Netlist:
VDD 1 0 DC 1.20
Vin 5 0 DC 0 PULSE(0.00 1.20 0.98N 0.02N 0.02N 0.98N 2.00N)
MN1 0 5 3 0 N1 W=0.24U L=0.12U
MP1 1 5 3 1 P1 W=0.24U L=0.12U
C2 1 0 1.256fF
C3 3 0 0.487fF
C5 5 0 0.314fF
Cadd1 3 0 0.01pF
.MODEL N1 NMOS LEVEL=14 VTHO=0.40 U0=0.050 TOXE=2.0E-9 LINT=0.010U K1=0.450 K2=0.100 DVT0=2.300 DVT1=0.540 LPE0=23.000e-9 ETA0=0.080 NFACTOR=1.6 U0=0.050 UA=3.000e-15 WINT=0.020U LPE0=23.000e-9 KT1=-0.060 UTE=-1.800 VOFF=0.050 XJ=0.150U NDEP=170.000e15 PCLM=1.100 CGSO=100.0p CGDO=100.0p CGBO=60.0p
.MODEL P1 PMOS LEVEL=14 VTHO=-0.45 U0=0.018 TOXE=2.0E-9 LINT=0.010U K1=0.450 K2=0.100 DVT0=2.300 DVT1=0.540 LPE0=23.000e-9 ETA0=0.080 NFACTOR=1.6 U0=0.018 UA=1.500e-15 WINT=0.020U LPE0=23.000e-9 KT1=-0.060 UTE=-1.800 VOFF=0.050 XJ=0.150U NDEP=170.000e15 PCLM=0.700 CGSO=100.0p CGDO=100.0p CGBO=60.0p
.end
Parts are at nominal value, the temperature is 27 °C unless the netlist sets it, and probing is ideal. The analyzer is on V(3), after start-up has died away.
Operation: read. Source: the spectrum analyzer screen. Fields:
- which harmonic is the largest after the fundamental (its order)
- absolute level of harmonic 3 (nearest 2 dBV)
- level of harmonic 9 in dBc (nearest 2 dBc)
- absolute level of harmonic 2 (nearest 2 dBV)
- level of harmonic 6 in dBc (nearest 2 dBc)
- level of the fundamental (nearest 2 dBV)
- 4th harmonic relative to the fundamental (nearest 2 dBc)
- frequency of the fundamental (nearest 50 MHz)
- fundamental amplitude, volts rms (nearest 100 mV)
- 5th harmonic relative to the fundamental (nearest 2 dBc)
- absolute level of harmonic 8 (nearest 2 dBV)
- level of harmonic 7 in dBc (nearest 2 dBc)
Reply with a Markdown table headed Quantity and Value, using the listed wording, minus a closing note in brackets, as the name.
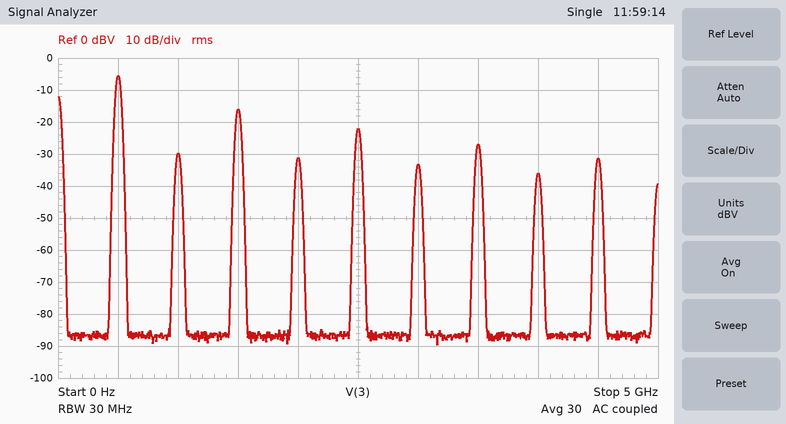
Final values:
| Quantity | Value |
|---|---|
| which harmonic is the largest after the fundamental | 3 |
| absolute level of harmonic 3 | -16 dBV |
| level of harmonic 9 in dBc | -26 dBc |
| absolute level of harmonic 2 | -30 dBV |
| level of harmonic 6 in dBc | -28 dBc |
| level of the fundamental | -6 dBV |
| 4th harmonic relative to the fundamental | -26 dBc |
| frequency of the fundamental | 500 MHz |
| fundamental amplitude, volts rms | 500 mV |
| 5th harmonic relative to the fundamental | -16 dBc |
| absolute level of harmonic 8 | -36 dBV |
| level of harmonic 7 in dBc | -22 dBc |
